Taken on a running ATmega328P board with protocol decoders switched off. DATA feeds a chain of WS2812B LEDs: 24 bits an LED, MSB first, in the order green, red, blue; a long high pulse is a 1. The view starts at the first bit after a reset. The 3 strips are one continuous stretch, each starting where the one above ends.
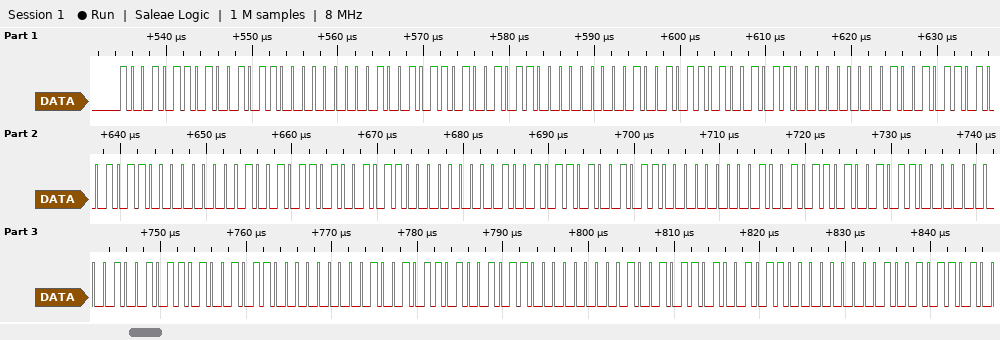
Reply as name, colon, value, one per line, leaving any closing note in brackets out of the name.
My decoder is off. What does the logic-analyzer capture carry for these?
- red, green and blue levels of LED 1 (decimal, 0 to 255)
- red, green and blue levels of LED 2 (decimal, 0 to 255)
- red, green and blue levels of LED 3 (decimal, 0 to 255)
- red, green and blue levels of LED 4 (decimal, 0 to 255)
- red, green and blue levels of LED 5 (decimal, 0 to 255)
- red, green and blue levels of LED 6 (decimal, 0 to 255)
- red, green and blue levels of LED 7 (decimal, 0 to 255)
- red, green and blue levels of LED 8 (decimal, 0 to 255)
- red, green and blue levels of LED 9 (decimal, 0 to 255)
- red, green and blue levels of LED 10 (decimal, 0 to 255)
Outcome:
red, green and blue levels of LED 1: 150, 150, 0
red, green and blue levels of LED 2: 150, 150, 0
red, green and blue levels of LED 3: 150, 150, 0
red, green and blue levels of LED 4: 150, 150, 0
red, green and blue levels of LED 5: 150, 150, 0
red, green and blue levels of LED 6: 150, 150, 0
red, green and blue levels of LED 7: 150, 150, 0
red, green and blue levels of LED 8: 150, 150, 0
red, green and blue levels of LED 9: 150, 150, 0
red, green and blue levels of LED 10: 150, 150, 0
